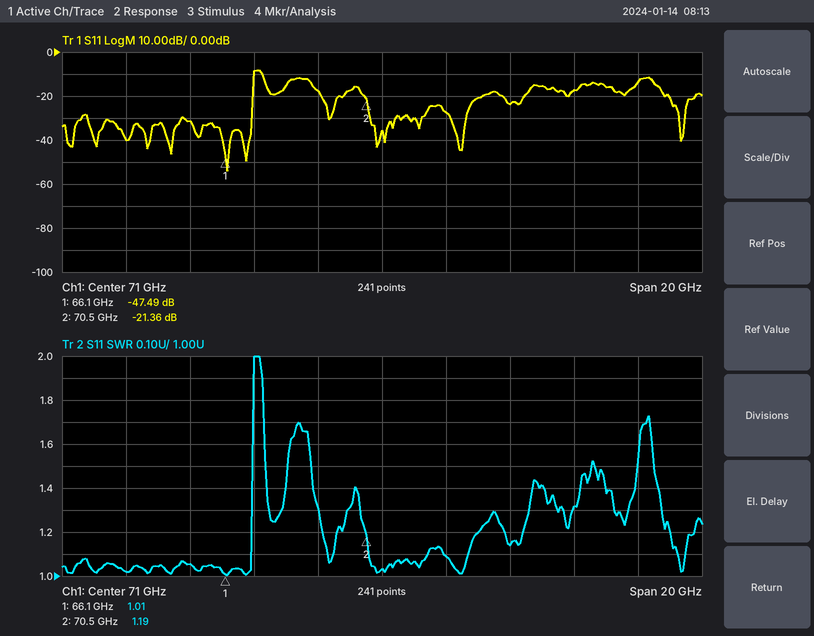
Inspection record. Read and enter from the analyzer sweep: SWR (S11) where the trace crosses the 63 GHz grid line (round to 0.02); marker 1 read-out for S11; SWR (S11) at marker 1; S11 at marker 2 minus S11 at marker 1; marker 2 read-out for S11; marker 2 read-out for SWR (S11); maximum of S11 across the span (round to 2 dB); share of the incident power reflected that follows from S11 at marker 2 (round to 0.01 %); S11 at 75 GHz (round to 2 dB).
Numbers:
1.02
-47.49 dB
1.01
26.13 dB
-21.36 dB
1.19
-8 dB
0.73 %
-24 dB
